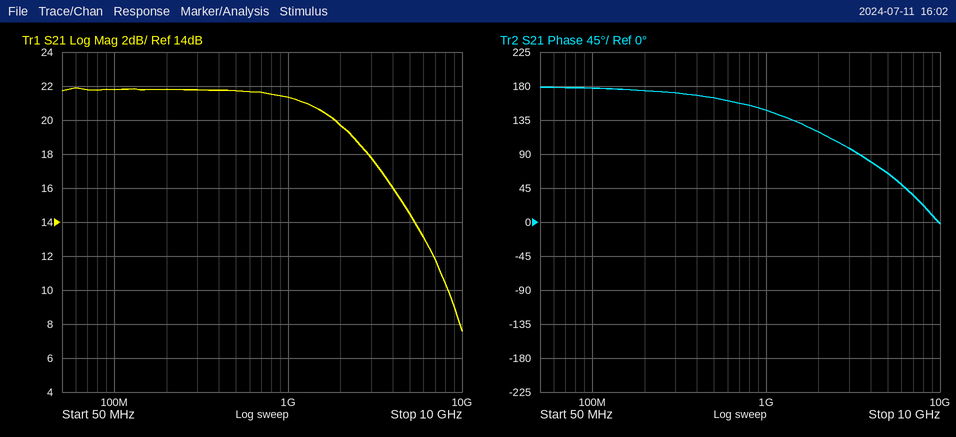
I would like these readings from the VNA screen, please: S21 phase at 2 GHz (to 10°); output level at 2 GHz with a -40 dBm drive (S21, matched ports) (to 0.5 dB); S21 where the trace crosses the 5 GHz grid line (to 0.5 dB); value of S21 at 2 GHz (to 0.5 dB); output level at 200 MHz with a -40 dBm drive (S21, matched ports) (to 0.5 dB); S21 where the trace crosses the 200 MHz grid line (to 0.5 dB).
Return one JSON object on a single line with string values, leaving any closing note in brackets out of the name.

{"S21 phase at 2 GHz": "120°", "output level at 2 GHz with a -40 dBm drive (S21, matched ports)": "-20.5 dBm", "S21 where the trace crosses the 5 GHz grid line": "14.5 dB", "value of S21 at 2 GHz": "19.5 dB", "output level at 200 MHz with a -40 dBm drive (S21, matched ports)": "-18.0 dBm", "S21 where the trace crosses the 200 MHz grid line": "22.0 dB"}
